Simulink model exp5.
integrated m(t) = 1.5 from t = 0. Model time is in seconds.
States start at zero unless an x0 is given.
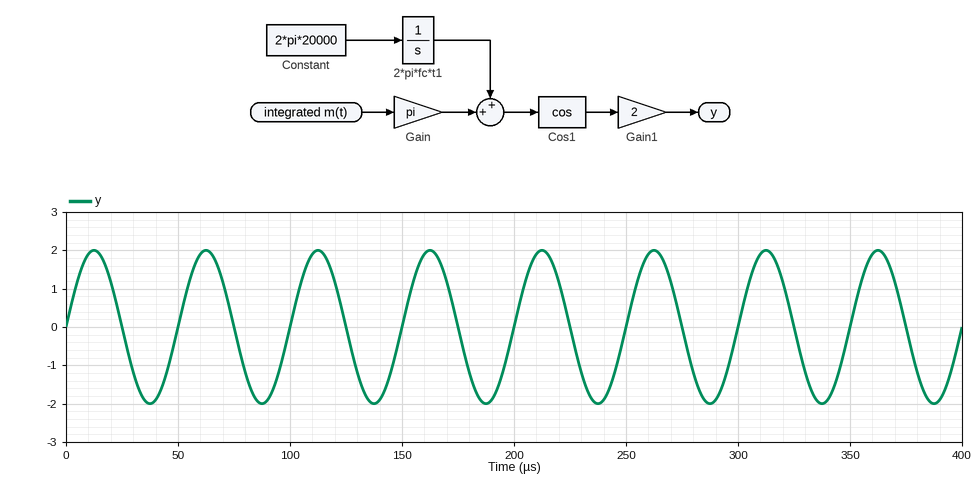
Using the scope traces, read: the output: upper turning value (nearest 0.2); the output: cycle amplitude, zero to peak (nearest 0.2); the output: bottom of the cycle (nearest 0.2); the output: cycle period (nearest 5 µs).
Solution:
2.0
2.0
-2.0
50 µs
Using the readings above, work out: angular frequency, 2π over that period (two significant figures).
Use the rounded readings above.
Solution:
0.13 rad/µs
